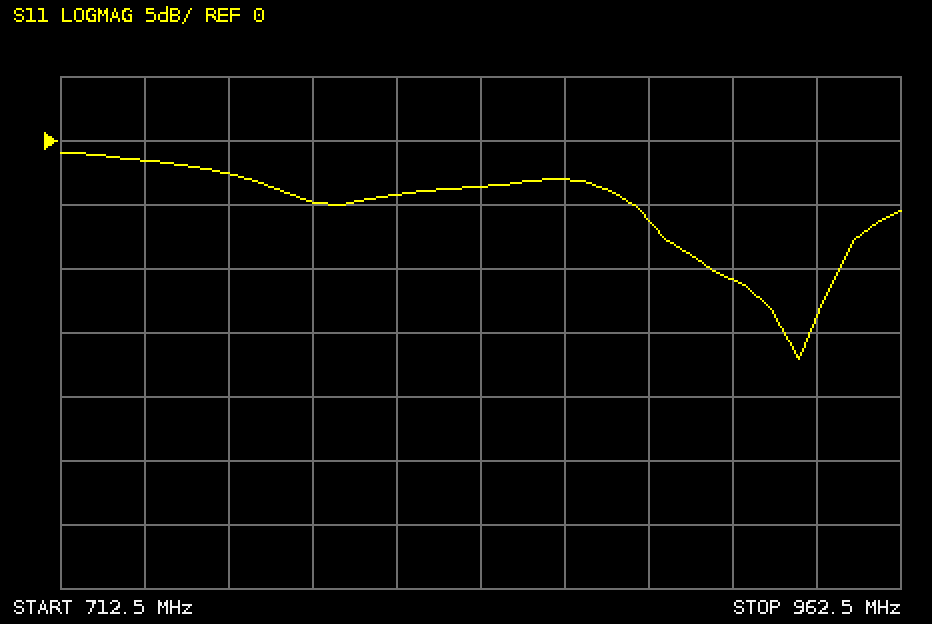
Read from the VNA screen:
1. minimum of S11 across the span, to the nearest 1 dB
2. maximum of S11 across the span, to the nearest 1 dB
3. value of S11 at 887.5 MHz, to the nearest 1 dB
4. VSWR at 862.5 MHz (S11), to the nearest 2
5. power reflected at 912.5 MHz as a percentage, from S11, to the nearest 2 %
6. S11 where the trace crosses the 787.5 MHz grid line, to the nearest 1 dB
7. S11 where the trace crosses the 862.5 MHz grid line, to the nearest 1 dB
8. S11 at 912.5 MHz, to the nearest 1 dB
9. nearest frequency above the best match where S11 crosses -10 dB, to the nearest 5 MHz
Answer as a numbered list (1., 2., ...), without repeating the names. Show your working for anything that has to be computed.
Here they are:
1. -17 dB
2. -1 dB
3. -6 dB
4. |Γ| = 10^(-3/20) = 0.7079; VSWR = (1 + 0.7079)/(1 − 0.7079) ≈ 6
5. 10^(-11/10) ≈ 8 %
6. -5 dB
7. -3 dB
8. -11 dB
9. 945 MHz
